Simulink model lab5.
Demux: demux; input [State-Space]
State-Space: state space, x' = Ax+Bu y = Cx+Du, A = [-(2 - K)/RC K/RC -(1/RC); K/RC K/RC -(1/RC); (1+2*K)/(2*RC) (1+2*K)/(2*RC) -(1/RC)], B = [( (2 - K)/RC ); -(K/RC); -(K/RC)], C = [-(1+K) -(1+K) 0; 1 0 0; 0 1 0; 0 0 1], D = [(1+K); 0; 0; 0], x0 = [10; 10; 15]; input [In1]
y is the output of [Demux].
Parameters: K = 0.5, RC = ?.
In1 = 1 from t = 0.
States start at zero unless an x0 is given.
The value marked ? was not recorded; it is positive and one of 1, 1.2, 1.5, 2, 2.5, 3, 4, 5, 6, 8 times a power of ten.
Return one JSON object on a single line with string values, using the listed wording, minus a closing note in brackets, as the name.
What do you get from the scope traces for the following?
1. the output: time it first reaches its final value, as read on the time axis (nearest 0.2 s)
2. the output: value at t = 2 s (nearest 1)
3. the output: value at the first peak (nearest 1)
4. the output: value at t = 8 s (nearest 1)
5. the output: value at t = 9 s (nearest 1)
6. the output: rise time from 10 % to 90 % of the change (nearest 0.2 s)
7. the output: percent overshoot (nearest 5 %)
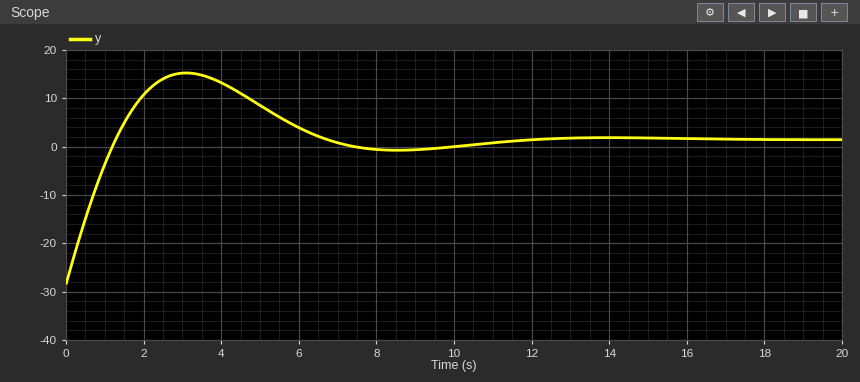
{"the output: time it first reaches its final value, as read on the time axis": "1.2 s", "the output: value at t = 2 s": "11", "the output: value at the first peak": "15", "the output: value at t = 8 s": "-1", "the output: value at t = 9 s": "-1", "the output: rise time from 10 % to 90 % of the change": "1.0 s", "the output: percent overshoot": "45 %"}
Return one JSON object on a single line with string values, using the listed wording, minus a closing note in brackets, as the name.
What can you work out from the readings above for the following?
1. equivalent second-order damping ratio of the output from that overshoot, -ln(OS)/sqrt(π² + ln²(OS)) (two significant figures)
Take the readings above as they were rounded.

{"equivalent second-order damping ratio of the output from that overshoot, -ln(OS)/sqrt(π² + ln²(OS))": "0.25"}
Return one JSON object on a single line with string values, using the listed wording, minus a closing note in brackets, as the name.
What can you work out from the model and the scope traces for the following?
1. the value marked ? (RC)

{"the value marked ?": "1.5"}
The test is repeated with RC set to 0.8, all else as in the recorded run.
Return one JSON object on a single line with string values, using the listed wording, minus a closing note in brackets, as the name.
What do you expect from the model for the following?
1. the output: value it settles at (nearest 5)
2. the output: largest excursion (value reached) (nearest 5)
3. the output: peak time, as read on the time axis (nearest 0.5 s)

{"the output: value it settles at": "0", "the output: largest excursion (value reached)": "15", "the output: peak time, as read on the time axis": "1.5 s"}
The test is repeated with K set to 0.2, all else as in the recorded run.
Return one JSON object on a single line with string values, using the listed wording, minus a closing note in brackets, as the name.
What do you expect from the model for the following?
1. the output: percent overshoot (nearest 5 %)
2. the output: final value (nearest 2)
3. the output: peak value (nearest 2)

{"the output: percent overshoot": "30 %", "the output: final value": "2", "the output: peak value": "8"}
